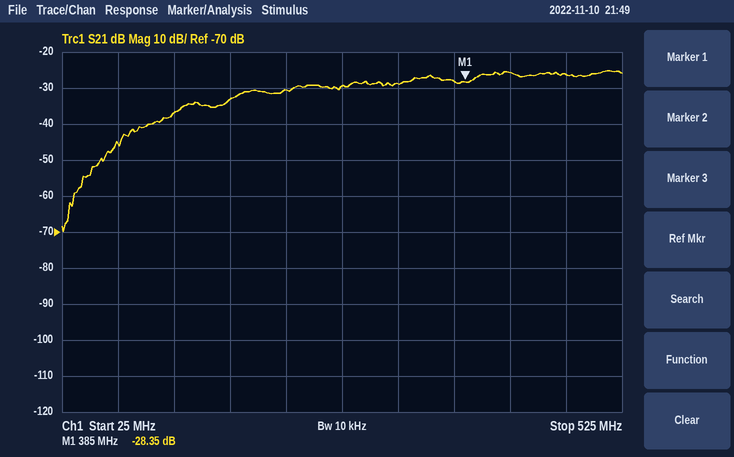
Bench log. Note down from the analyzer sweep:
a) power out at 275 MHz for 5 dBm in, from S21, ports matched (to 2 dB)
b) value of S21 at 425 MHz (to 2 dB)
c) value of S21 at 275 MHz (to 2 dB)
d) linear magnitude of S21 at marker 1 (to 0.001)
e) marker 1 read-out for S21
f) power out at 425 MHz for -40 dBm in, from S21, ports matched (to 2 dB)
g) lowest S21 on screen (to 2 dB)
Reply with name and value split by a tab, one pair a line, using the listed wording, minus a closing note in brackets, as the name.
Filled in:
power out at 275 MHz for 5 dBm in, from S21, ports matched	-24 dBm
value of S21 at 425 MHz	-26 dB
value of S21 at 275 MHz	-30 dB
linear magnitude of S21 at marker 1	0.038
marker 1 read-out for S21	-28.35 dB
power out at 425 MHz for -40 dBm in, from S21, ports matched	-66 dBm
lowest S21 on screen	-70 dB
